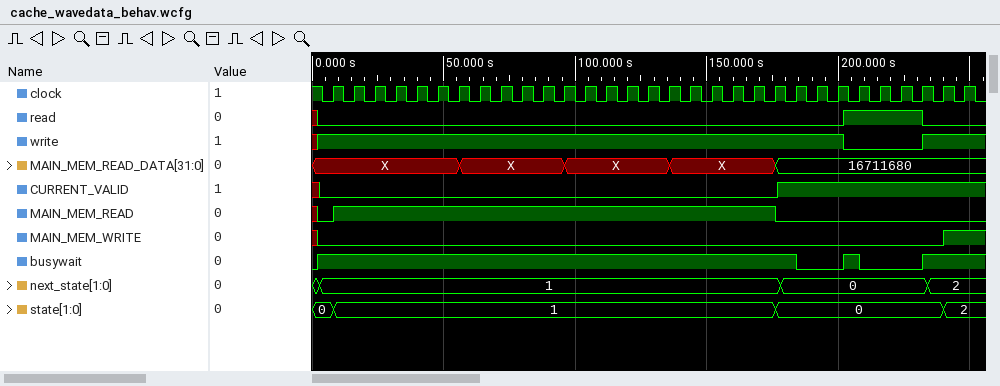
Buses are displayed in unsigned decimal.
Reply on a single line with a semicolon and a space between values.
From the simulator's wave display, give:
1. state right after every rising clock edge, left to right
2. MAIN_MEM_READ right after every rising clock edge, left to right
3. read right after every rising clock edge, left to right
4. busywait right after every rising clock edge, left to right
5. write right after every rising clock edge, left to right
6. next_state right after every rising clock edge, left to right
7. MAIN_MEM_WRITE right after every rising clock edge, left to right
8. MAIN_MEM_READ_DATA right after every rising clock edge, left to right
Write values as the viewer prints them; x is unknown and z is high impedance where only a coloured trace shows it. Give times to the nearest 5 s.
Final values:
1, 1, 1, 1, 1, 1, 1, 1, 1, 1, 1, 1, 1, 1, 1, 1, 1, 1, 1, 1, 1, 0, 0, 0, 0, 0, 0, 0, 0, 2, 2; 1 1 1 1 1 1 1 1 1 1 1 1 1 1 1 1 1 1 1 1 1 0 0 0 0 0 0 0 0 0 0; 0 0 0 0 0 0 0 0 0 0 0 0 0 0 0 0 0 0 0 0 0 0 0 0 0 1 1 1 0 0 0; 1 1 1 1 1 1 1 1 1 1 1 1 1 1 1 1 1 1 1 1 1 1 0 0 0 0 0 0 1 1 1; 1 1 1 1 1 1 1 1 1 1 1 1 1 1 1 1 1 1 1 1 1 1 1 1 1 0 0 0 1 1 1; 1, 1, 1, 1, 1, 1, 1, 1, 1, 1, 1, 1, 1, 1, 1, 1, 1, 1, 1, 1, 1, 1, 0, 0, 0, 0, 0, 0, 0, 2, 2; 0 0 0 0 0 0 0 0 0 0 0 0 0 0 0 0 0 0 0 0 0 0 0 0 0 0 0 0 0 1 1; X, X, X, X, X, X, X, X, X, X, X, X, X, X, X, X, X, X, X, X, X, 16711680, 16711680, 16711680, 16711680, 16711680, 16711680, 16711680, 16711680, 16711680, 16711680
